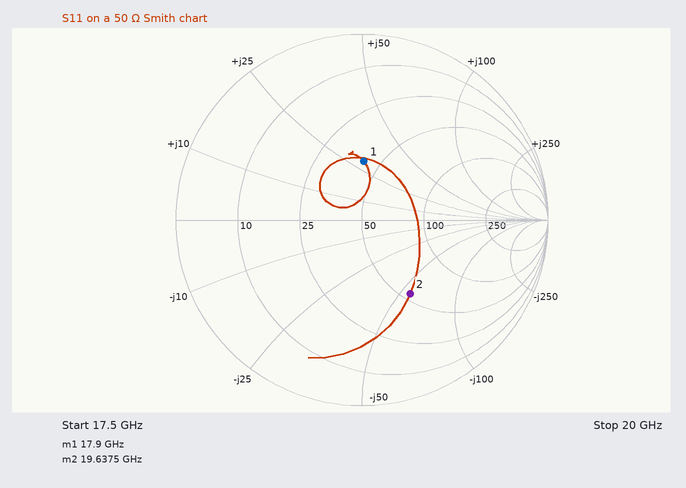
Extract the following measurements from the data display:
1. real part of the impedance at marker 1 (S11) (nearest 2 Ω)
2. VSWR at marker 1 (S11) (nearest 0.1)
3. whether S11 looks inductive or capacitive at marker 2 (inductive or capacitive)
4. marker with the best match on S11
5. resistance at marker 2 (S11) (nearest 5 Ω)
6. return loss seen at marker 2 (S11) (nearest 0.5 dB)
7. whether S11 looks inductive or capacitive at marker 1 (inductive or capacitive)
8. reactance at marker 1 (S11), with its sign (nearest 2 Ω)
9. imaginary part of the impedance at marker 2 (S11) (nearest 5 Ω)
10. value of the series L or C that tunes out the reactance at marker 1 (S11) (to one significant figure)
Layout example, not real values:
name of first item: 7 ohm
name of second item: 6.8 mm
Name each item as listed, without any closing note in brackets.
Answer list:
real part of the impedance at marker 1 (S11): 42 Ω
VSWR at marker 1 (S11): 1.9
whether S11 looks inductive or capacitive at marker 2: capacitive
marker with the best match on S11: marker 1
resistance at marker 2 (S11): 55 Ω
return loss seen at marker 2 (S11): 6.5 dB
whether S11 looks inductive or capacitive at marker 1: inductive
reactance at marker 1 (S11), with its sign: +30 Ω
imaginary part of the impedance at marker 2 (S11): -55 Ω
value of the series L or C that tunes out the reactance at marker 1 (S11): 300 fF
